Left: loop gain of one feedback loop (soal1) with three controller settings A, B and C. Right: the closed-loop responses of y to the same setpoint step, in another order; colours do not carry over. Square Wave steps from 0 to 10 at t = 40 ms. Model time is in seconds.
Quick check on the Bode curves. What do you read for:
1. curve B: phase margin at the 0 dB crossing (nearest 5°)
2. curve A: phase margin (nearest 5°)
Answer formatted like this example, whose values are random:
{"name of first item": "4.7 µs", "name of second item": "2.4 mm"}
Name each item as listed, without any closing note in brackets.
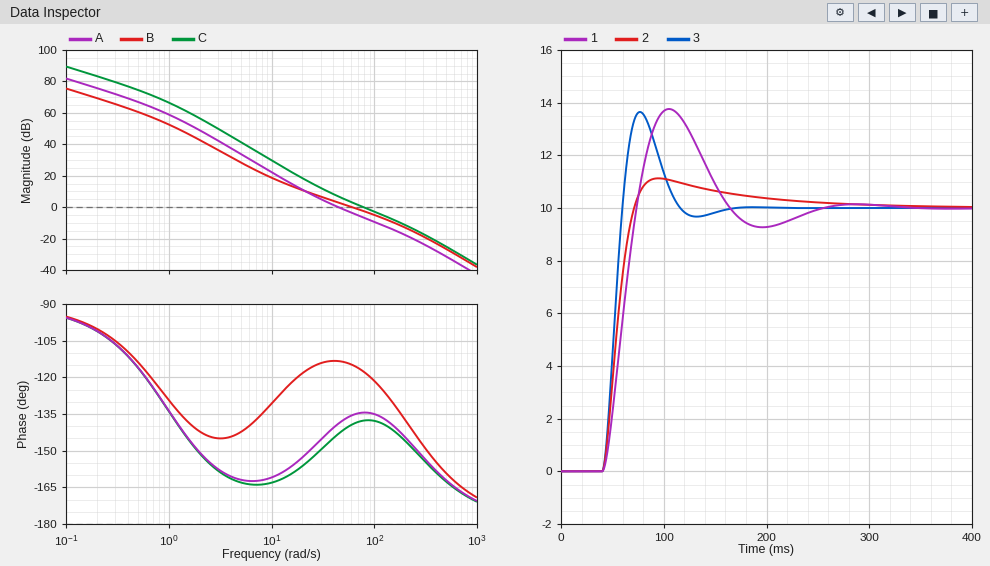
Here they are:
{"curve B: phase margin at the 0 dB crossing": "65°", "curve A: phase margin": "40°"}
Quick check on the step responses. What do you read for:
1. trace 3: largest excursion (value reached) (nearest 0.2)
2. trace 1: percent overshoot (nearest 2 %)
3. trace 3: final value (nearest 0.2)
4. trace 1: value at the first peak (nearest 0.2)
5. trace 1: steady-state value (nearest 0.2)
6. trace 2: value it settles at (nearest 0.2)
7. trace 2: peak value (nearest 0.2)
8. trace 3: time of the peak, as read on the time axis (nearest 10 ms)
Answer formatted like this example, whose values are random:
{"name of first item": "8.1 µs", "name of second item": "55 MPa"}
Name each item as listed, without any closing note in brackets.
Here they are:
{"trace 3: largest excursion (value reached)": "13.6", "trace 1: percent overshoot": "38 %", "trace 3: final value": "10.0", "trace 1: value at the first peak": "13.8", "trace 1: steady-state value": "10.0", "trace 2: value it settles at": "10.0", "trace 2: peak value": "11.2", "trace 3: time of the peak, as read on the time axis": "80 ms"}
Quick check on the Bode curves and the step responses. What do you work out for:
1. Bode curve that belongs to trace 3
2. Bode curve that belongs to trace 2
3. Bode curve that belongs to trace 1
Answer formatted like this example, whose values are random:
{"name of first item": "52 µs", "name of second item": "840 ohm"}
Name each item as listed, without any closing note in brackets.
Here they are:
{"Bode curve that belongs to trace 3": "C", "Bode curve that belongs to trace 2": "B", "Bode curve that belongs to trace 1": "A"}
